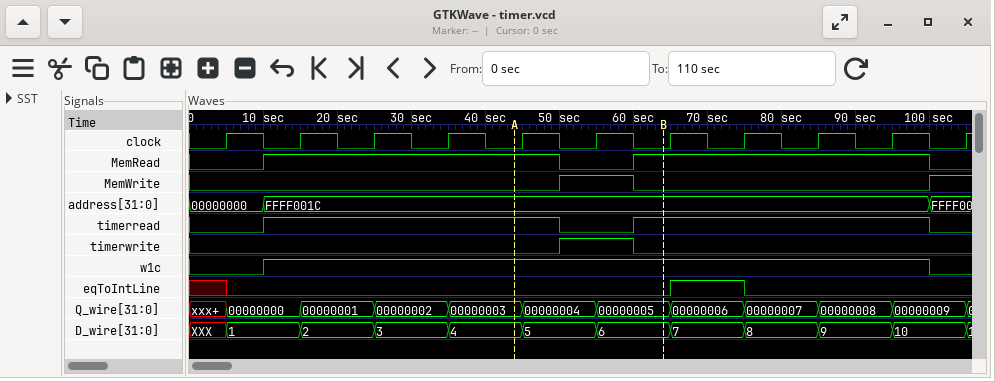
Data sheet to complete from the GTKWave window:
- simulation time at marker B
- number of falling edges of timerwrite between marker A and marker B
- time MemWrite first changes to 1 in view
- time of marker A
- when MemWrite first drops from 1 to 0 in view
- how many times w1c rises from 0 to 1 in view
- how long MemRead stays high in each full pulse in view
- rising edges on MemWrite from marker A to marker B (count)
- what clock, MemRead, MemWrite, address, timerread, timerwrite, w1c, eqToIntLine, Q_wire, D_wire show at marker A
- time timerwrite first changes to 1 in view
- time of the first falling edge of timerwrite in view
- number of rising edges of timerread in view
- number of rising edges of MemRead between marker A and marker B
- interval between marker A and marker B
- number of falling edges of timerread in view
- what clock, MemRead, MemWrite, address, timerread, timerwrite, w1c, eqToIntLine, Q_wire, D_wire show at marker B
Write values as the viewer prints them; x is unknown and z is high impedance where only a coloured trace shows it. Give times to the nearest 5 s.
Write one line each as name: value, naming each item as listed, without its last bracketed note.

simulation time at marker B: 65 s
number of falling edges of timerwrite between marker A and marker B: 1
time MemWrite first changes to 1 in view: 50 s
time of marker A: 45 s
when MemWrite first drops from 1 to 0 in view: 60 s
how many times w1c rises from 0 to 1 in view: 1
how long MemRead stays high in each full pulse in view: 40 s, 40 s
rising edges on MemWrite from marker A to marker B: 1
what clock, MemRead, MemWrite, address, timerread, timerwrite, w1c, eqToIntLine, Q_wire, D_wire show at marker A: clock=0, MemRead=1, MemWrite=0, address=FFFF001C, timerread=1, timerwrite=0, w1c=1, eqToIntLine=0, Q_wire=00000003, D_wire=4
time timerwrite first changes to 1 in view: 50 s
time of the first falling edge of timerwrite in view: 60 s
number of rising edges of timerread in view: 2
number of rising edges of MemRead between marker A and marker B: 1
interval between marker A and marker B: 20 s
number of falling edges of timerread in view: 2
what clock, MemRead, MemWrite, address, timerread, timerwrite, w1c, eqToIntLine, Q_wire, D_wire show at marker B: clock=0, MemRead=1, MemWrite=0, address=FFFF001C, timerread=1, timerwrite=0, w1c=1, eqToIntLine=0, Q_wire=00000005, D_wire=6
